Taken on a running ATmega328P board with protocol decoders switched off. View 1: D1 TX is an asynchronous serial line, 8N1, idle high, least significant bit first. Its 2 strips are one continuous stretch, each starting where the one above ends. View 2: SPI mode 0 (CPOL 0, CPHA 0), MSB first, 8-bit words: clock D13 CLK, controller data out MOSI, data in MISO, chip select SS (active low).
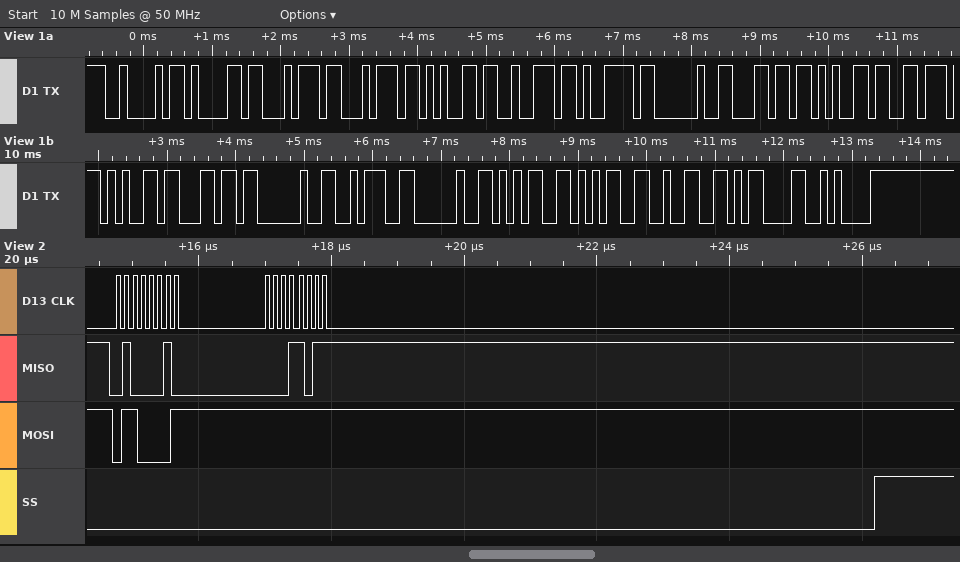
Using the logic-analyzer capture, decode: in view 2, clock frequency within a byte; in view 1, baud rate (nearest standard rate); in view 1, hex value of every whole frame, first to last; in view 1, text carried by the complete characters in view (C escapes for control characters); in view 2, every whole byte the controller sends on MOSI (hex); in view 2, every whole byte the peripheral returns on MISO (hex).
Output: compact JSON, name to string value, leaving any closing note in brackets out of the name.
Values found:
{"in view 2, clock frequency within a byte": "8 MHz", "in view 1, baud rate": "9600 baud", "in view 1, hex value of every whole frame, first to last": "0x42 0x61 0x74 0x74 0x65 0x72 0x79 0x20 0x6C 0x65 0x76 0x65 0x6C 0x20 0x3A 0x20 0x35 0x35 0x32 0x0D 0x0A", "in view 1, text carried by the complete characters in view": "\"Battery level : 552\\r\\n\"", "in view 2, every whole byte the controller sends on MOSI": "61 FF", "in view 2, every whole byte the peripheral returns on MISO": "42 1B"}
